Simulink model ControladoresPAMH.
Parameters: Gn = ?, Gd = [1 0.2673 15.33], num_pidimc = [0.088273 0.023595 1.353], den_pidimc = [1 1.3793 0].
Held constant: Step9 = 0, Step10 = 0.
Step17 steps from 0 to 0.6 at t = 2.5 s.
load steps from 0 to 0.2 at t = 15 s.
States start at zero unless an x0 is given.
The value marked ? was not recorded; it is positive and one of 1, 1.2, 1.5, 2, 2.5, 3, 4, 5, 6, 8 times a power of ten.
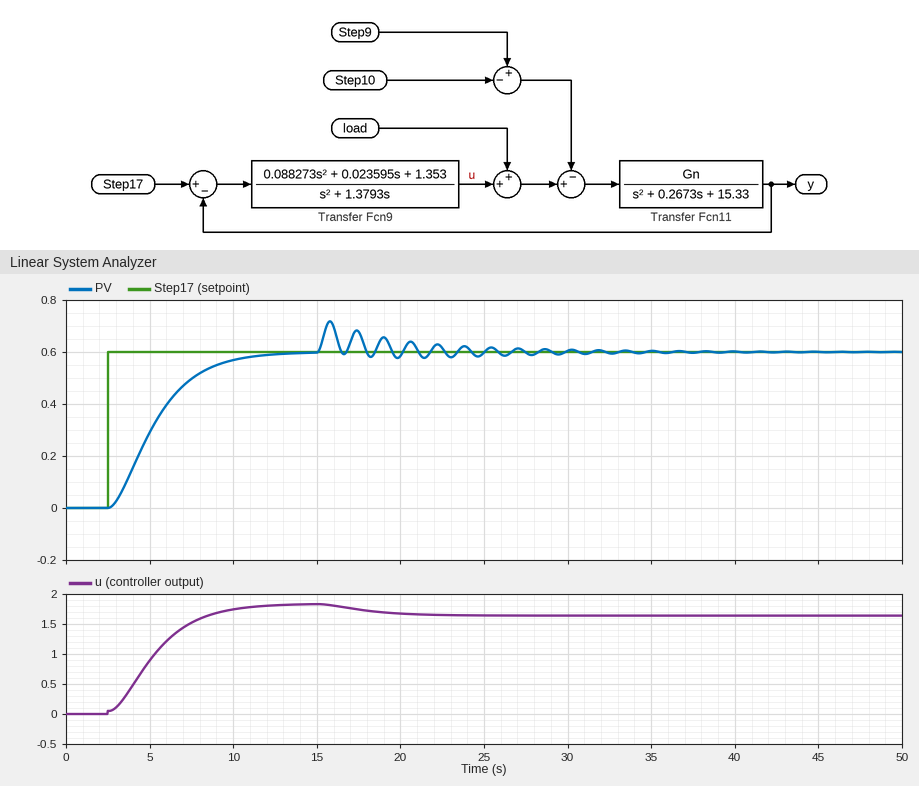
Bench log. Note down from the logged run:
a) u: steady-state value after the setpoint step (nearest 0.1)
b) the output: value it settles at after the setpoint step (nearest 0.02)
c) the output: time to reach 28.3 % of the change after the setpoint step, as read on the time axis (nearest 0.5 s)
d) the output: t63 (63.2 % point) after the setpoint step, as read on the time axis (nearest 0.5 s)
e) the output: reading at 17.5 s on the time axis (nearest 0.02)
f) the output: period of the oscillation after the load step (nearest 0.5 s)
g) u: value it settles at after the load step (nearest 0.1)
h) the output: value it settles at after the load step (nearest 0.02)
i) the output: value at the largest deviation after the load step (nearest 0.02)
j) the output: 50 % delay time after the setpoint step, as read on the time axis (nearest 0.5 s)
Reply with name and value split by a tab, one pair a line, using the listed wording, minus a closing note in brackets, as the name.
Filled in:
u: steady-state value after the setpoint step	1.8
the output: value it settles at after the setpoint step	0.60
the output: time to reach 28.3 % of the change after the setpoint step, as read on the time axis	4.0 s
the output: t63 (63.2 % point) after the setpoint step, as read on the time axis	6.0 s
the output: reading at 17.5 s on the time axis	0.68
the output: period of the oscillation after the load step	1.5 s
u: value it settles at after the load step	1.6
the output: value it settles at after the load step	0.60
the output: value at the largest deviation after the load step	0.72
the output: 50 % delay time after the setpoint step, as read on the time axis	5.0 s
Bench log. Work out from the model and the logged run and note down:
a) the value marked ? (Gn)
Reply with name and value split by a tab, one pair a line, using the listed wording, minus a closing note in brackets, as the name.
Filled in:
the value marked ?	5
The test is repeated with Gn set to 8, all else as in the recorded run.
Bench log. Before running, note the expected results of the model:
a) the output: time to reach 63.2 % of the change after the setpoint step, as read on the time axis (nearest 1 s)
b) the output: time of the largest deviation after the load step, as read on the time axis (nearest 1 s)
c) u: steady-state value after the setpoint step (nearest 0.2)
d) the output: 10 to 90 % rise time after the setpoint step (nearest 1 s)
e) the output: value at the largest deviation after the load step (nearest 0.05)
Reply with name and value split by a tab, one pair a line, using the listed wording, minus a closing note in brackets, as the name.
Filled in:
the output: time to reach 63.2 % of the change after the setpoint step, as read on the time axis	5 s
the output: time of the largest deviation after the load step, as read on the time axis	16 s
u: steady-state value after the setpoint step	1.2
the output: 10 to 90 % rise time after the setpoint step	3 s
the output: value at the largest deviation after the load step	0.80
